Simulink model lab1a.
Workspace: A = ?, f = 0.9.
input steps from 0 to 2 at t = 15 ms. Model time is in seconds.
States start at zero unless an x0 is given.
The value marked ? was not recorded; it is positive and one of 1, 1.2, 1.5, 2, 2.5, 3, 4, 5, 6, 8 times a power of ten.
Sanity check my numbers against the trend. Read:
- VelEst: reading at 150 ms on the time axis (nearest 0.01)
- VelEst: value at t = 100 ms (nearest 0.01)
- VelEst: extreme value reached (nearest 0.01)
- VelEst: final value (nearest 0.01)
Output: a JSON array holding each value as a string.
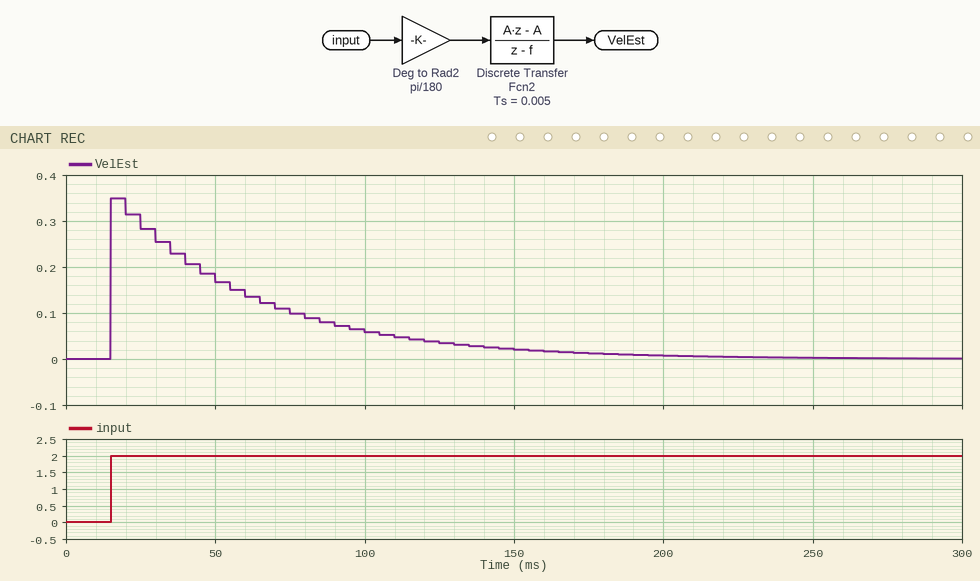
["0.02", "0.06", "0.35", "0.00"]
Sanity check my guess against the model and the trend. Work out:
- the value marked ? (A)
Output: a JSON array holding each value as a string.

["10"]
